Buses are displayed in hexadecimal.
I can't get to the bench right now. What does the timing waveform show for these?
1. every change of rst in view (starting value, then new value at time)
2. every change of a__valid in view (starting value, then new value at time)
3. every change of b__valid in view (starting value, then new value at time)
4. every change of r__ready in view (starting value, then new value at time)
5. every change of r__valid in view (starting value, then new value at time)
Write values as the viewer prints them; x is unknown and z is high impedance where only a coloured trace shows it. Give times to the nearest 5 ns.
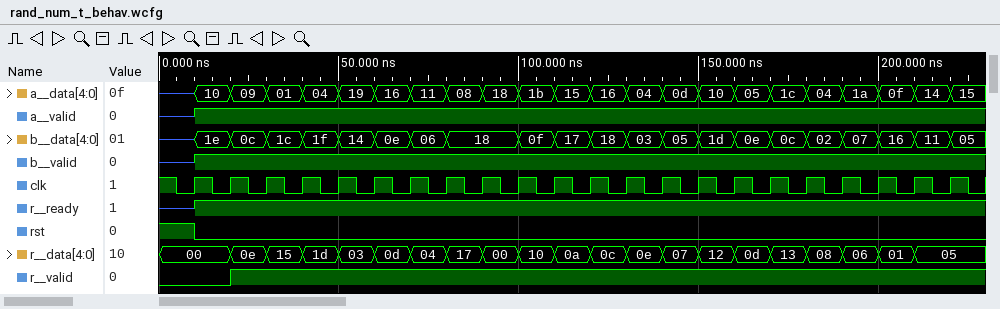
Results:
1, 0 at 10 ns
z, 1 at 10 ns
z, 1 at 10 ns
z, 1 at 10 ns
0, 1 at 20 ns
